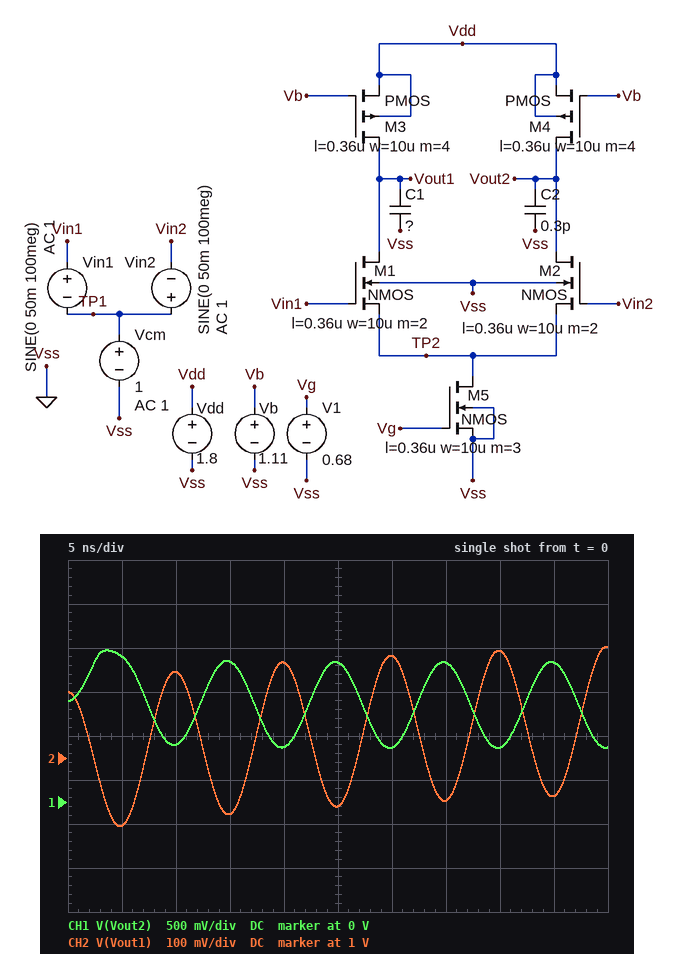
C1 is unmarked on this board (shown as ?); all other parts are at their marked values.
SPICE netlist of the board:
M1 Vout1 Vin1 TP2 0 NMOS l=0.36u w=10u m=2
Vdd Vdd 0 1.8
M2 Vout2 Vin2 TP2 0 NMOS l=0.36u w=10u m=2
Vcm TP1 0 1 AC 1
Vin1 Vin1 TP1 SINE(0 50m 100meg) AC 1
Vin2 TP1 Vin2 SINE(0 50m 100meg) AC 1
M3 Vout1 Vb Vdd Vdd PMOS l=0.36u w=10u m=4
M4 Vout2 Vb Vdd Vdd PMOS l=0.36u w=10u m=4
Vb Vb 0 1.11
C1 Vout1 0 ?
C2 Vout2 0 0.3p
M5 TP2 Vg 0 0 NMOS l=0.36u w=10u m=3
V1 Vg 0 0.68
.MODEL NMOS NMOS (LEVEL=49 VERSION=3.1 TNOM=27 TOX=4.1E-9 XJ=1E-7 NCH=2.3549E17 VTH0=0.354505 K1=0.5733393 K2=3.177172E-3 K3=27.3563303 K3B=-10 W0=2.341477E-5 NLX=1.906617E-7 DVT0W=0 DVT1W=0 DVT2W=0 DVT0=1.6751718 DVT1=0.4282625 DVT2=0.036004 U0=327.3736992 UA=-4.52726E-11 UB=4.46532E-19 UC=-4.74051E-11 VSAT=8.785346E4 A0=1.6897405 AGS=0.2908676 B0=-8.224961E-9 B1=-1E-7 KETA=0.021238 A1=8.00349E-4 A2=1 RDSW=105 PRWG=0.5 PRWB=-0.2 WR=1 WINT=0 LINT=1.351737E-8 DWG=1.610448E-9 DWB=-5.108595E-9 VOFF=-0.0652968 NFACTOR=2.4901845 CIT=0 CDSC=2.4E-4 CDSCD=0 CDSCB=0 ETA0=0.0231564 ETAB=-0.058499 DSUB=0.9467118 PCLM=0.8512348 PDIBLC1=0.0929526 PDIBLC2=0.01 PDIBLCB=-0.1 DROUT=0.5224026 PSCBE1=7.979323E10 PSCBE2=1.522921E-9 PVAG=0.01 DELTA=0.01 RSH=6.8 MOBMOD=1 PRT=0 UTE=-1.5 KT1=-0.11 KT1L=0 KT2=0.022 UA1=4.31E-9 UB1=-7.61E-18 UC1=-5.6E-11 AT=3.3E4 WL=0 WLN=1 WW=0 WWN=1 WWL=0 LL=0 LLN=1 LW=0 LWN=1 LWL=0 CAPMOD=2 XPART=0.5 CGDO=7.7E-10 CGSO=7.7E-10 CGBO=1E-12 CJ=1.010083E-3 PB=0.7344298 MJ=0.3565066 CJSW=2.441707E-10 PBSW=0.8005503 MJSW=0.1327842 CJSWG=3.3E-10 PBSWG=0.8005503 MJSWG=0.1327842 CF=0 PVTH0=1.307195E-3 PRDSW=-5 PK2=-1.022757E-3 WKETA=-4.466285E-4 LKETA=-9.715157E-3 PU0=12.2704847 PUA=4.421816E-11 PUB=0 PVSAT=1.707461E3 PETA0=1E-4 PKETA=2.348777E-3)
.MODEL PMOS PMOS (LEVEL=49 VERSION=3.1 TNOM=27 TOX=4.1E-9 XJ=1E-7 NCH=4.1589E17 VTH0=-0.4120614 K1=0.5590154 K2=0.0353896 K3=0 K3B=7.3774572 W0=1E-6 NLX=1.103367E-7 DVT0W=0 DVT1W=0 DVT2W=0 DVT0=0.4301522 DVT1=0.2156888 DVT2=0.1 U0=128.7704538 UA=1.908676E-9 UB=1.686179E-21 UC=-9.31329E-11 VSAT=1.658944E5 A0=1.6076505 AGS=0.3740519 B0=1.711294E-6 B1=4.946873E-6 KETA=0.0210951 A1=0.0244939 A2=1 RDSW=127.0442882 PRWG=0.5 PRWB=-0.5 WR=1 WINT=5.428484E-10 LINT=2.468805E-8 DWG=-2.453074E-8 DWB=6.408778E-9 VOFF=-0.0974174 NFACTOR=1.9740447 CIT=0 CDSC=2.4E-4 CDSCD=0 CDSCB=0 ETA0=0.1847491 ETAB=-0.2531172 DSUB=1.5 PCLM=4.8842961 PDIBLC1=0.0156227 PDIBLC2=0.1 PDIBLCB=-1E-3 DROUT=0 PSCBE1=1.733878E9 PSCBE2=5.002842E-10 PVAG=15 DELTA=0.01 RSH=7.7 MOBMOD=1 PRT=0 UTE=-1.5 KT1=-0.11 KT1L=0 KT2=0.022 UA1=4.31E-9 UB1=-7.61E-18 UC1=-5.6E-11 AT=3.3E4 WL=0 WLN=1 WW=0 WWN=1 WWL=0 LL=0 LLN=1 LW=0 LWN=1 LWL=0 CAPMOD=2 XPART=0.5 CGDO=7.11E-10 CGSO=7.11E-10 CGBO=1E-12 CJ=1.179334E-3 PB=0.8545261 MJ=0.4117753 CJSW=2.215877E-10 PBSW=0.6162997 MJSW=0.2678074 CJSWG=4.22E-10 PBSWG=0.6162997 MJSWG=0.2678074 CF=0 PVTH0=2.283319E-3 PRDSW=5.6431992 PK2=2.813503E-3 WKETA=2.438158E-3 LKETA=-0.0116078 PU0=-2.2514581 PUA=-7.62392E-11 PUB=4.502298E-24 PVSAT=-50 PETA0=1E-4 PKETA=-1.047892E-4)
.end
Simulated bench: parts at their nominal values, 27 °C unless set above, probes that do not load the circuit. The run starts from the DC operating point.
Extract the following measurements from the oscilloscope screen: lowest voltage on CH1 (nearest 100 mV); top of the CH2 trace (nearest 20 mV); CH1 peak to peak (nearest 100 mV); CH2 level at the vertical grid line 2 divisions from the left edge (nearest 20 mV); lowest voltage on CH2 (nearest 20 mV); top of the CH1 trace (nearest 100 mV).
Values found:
600 mV
1.26 V
1.1 V
1.20 V
840 mV
1.7 V
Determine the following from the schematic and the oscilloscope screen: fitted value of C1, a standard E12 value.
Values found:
1 pF
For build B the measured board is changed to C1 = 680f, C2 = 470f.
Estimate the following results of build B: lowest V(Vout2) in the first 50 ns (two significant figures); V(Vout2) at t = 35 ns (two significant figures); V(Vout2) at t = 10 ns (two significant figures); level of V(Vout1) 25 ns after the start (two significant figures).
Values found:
800 mV
1.5 V
920 mV
830 mV
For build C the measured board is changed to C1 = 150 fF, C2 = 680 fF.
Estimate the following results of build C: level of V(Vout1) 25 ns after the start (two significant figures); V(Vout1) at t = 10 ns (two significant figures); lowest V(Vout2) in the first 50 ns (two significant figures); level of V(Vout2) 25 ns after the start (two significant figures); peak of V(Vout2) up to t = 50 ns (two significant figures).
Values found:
420 mV
1.6 V
650 mV
1.2 V
1.4 V
